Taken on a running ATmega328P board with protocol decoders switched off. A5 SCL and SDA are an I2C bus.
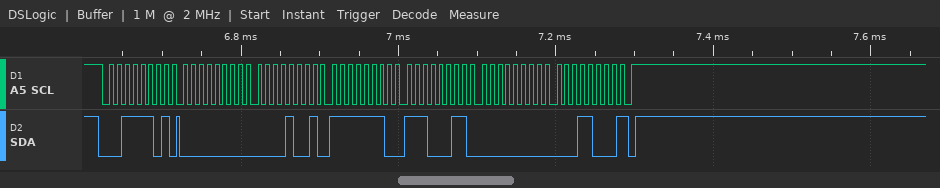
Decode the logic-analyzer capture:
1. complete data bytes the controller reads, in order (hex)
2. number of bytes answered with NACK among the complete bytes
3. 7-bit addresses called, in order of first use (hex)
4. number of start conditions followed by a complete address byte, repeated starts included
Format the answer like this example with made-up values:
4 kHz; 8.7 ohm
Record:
00 09 FE E3 00 18; 1; 0x1E; 1
